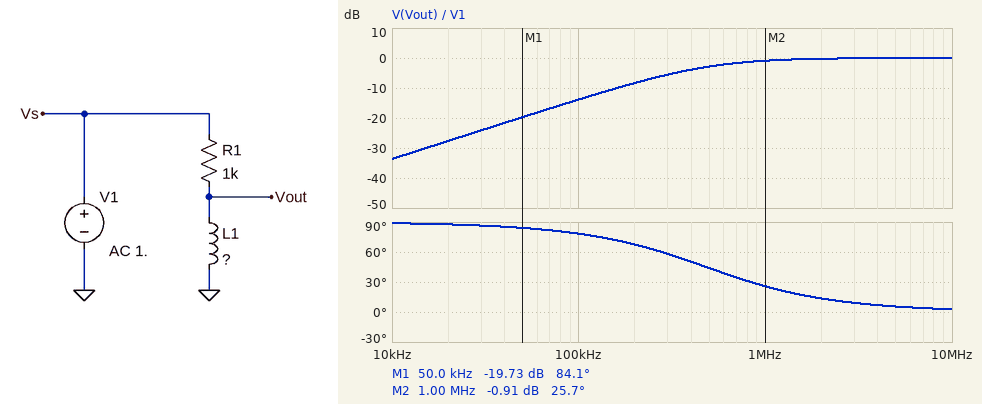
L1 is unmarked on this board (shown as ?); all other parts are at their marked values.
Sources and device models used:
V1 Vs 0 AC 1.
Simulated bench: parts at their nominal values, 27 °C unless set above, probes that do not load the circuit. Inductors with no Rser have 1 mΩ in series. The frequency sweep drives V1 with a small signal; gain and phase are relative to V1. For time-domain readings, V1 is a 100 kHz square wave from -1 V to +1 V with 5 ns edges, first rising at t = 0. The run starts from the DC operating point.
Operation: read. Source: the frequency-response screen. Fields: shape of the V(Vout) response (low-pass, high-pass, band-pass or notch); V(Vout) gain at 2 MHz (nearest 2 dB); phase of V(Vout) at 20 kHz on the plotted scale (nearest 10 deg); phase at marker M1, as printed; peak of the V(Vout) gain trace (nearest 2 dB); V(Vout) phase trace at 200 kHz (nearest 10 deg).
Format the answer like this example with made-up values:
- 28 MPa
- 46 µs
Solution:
- high-pass
- 0 dB
- 90 deg
- 84.1 deg
- 0 dB
- 70 deg
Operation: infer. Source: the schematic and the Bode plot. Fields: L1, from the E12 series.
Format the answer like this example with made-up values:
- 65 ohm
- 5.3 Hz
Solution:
- 330 µH
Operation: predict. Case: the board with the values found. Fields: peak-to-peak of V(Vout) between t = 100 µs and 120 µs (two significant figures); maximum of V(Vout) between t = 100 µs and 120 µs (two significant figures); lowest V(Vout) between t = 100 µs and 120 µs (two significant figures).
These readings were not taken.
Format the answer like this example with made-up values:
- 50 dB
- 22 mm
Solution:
- 4.0 V
- 2.0 V
- -2.0 V
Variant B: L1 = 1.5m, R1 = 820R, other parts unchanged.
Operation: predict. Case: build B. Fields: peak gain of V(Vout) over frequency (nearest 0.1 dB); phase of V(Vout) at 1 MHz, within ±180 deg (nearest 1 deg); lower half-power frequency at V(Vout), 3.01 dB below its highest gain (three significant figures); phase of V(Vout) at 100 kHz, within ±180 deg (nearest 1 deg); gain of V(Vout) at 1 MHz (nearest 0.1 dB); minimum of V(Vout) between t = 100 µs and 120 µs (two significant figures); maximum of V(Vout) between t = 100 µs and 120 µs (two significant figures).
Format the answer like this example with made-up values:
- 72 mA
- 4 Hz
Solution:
- 0 dB
- 5 deg
- 87.0 kHz
- 41 deg
- 0 dB
- -1.9 V
- 1.9 V
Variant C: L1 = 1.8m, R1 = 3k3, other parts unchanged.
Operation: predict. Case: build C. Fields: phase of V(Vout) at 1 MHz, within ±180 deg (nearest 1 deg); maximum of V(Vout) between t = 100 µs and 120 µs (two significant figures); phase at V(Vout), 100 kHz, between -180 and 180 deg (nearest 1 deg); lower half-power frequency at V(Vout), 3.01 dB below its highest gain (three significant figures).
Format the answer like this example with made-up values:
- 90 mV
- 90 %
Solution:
- 16 deg
- 2.0 V
- 71 deg
- 292 kHz
